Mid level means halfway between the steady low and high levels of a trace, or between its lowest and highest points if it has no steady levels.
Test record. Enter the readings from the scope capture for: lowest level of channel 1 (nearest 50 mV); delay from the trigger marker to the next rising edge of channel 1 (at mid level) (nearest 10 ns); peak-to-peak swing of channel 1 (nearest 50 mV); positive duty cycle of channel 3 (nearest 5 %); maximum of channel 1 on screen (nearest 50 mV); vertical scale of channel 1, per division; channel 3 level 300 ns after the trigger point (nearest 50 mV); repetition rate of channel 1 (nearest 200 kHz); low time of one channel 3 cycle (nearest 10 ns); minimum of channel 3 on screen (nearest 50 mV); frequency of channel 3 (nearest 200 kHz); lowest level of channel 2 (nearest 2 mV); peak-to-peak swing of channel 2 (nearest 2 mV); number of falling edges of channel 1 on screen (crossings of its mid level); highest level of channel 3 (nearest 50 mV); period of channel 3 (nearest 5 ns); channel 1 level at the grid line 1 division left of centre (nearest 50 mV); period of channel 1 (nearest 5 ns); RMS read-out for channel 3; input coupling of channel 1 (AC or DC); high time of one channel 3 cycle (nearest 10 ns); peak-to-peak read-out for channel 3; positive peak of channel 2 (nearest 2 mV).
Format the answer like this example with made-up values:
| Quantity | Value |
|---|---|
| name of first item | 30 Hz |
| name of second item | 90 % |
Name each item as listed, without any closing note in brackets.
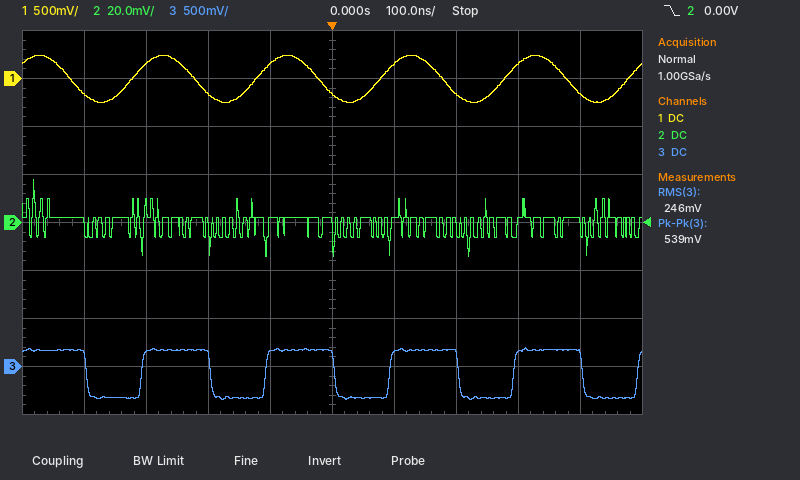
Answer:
| Quantity | Value |
|---|---|
| lowest level of channel 1 | -250 mV |
| delay from the trigger marker to the next rising edge of channel 1 (at mid level) | 80 ns |
| peak-to-peak swing of channel 1 | 500 mV |
| positive duty cycle of channel 3 | 55 % |
| maximum of channel 1 on screen | 250 mV |
| vertical scale of channel 1, per division | 500 mV |
| channel 3 level 300 ns after the trigger point | 100 mV |
| repetition rate of channel 1 | 5.0 MHz |
| low time of one channel 3 cycle | 90 ns |
| minimum of channel 3 on screen | -350 mV |
| frequency of channel 3 | 5.0 MHz |
| lowest level of channel 2 | -14 mV |
| peak-to-peak swing of channel 2 | 32 mV |
| number of falling edges of channel 1 on screen | 5 |
| highest level of channel 3 | 200 mV |
| period of channel 3 | 200 ns |
| channel 1 level at the grid line 1 division left of centre | 150 mV |
| period of channel 1 | 200 ns |
| RMS read-out for channel 3 | 246 mV |
| input coupling of channel 1 | DC |
| high time of one channel 3 cycle | 110 ns |
| peak-to-peak read-out for channel 3 | 539 mV |
| positive peak of channel 2 | 18 mV |
